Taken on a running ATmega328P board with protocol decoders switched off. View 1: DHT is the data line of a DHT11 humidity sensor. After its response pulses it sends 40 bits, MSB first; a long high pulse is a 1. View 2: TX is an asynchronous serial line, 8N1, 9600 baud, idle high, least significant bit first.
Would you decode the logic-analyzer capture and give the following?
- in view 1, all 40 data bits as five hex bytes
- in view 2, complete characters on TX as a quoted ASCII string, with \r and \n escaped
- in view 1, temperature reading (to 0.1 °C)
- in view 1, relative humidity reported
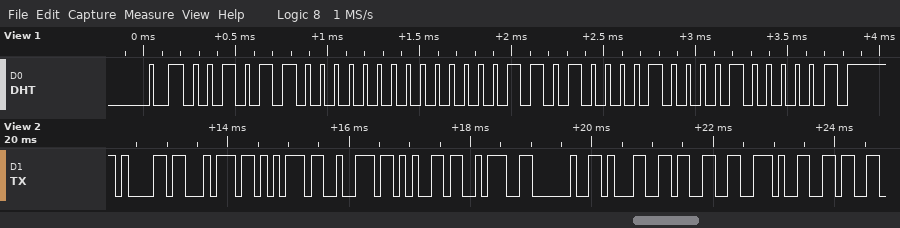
2C 00 0D 08 41
"ature: 13.6"
13.8 °C
44 %
